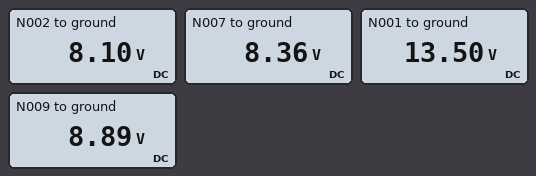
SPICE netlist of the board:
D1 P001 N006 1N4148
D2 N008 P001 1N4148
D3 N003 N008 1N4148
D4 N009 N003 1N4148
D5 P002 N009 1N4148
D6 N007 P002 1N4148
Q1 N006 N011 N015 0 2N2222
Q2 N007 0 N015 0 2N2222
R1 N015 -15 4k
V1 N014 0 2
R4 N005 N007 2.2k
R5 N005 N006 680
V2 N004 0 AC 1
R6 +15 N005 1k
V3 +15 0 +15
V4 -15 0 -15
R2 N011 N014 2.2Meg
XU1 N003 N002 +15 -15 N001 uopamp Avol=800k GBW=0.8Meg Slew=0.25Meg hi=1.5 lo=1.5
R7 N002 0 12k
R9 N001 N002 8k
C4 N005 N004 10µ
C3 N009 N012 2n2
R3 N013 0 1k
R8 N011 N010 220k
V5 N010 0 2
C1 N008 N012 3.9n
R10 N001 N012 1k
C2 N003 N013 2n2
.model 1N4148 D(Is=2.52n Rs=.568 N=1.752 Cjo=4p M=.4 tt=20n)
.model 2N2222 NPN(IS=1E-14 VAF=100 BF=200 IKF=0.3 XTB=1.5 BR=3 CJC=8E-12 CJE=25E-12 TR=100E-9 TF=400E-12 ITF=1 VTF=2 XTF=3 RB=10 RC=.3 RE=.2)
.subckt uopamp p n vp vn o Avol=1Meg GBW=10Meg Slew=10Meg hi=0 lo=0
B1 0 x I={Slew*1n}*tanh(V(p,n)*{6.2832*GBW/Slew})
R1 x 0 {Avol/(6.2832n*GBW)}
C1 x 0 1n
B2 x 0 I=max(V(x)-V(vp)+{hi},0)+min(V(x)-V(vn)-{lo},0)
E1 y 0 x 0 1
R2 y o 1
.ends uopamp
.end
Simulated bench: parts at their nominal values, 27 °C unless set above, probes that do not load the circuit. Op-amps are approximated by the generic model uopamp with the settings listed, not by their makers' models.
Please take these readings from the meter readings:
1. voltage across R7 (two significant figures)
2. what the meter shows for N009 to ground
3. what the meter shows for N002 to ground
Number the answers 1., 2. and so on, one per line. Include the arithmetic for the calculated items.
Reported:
1. 8.1 V = 8.1 V
2. 8.89 V
3. 8.10 V
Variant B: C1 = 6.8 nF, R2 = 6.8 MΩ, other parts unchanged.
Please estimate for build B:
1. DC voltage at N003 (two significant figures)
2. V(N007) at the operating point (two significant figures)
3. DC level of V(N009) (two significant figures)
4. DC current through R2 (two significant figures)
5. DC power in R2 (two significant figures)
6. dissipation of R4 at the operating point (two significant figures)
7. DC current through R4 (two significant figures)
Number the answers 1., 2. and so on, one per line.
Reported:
1. 9.1 V
2. 8.1 V
3. 8.7 V
4. 290 nA
5. 580 nW
6. 5.1 mW
7. 1.5 mA
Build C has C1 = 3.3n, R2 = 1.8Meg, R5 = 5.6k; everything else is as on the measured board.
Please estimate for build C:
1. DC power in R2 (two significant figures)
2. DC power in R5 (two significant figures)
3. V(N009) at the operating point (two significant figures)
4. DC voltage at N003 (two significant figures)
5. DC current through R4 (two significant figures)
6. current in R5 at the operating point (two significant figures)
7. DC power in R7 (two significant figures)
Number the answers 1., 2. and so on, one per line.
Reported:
1. 2.2 µW
2. 12 mW
3. 5.6 V
4. 5.1 V
5. 2.1 mA
6. 1.4 mA
7. 2.1 mW
